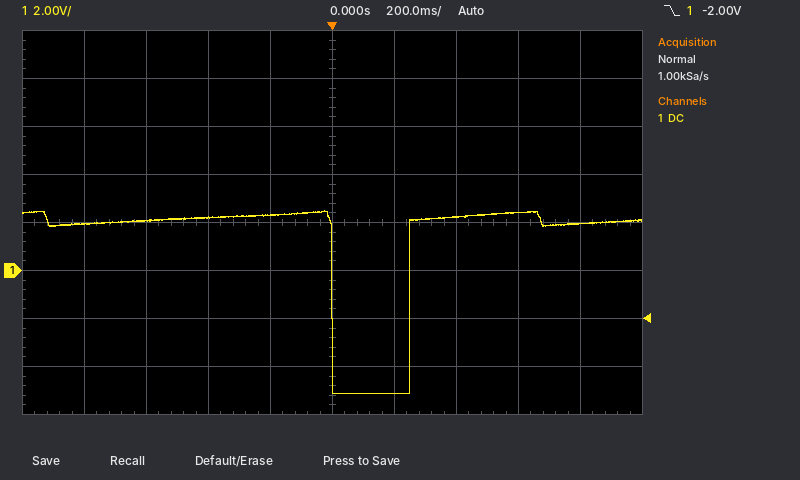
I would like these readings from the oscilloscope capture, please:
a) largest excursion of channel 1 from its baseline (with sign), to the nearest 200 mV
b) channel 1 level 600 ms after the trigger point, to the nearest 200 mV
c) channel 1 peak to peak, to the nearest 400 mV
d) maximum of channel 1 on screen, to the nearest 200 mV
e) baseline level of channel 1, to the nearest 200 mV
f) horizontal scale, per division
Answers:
-7.2 V
2.4 V
7.6 V
2.4 V
2.2 V
200 ms
